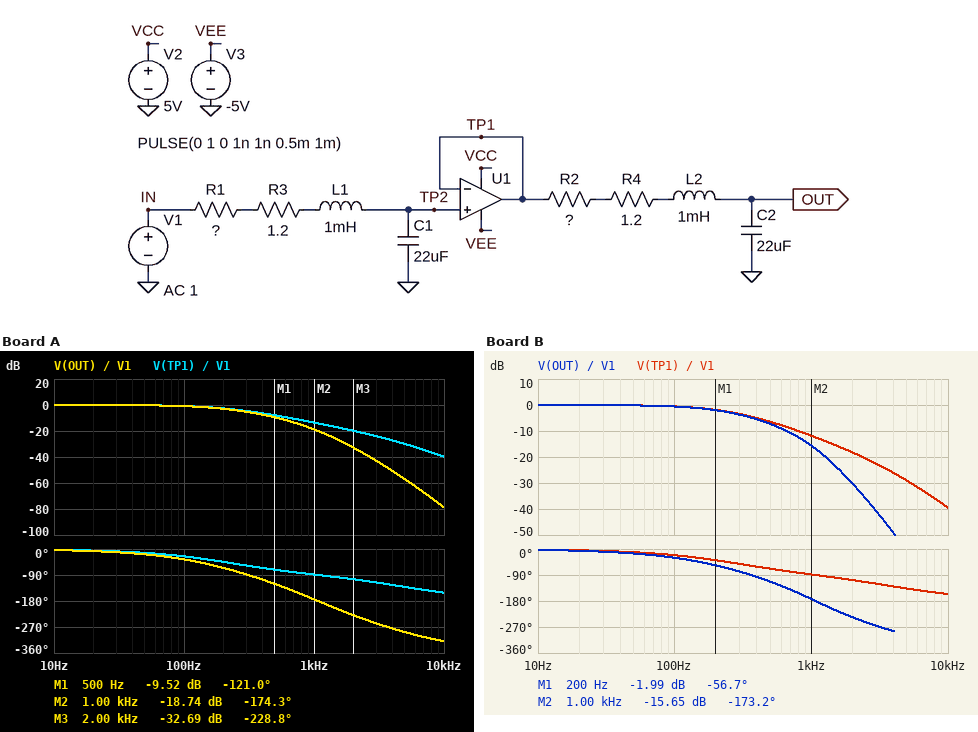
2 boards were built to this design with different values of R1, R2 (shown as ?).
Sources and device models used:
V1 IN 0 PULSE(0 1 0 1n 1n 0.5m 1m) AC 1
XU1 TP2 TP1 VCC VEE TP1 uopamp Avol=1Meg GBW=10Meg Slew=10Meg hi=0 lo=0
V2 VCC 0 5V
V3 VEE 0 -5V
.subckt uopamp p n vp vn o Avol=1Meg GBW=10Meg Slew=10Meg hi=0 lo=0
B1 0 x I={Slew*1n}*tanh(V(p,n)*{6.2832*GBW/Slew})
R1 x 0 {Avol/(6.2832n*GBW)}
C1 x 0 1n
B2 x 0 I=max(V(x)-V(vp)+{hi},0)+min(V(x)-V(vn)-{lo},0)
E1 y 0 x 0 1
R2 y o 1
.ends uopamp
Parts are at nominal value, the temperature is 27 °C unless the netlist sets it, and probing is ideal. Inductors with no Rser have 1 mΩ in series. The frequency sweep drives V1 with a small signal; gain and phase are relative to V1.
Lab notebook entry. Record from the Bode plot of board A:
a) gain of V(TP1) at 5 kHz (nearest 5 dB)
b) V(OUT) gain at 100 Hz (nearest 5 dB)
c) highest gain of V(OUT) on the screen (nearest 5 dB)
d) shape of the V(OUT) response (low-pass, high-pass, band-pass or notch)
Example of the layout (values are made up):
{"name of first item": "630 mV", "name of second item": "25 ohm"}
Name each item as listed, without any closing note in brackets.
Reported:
{"gain of V(TP1) at 5 kHz": "-30 dB", "V(OUT) gain at 100 Hz": "0 dB", "highest gain of V(OUT) on the screen": "0 dB", "shape of the V(OUT) response": "low-pass"}
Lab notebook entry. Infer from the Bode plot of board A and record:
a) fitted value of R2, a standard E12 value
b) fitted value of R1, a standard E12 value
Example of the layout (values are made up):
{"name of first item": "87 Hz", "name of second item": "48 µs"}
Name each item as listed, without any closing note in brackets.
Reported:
{"fitted value of R2, a standard E12 value": "12 Ω", "fitted value of R1, a standard E12 value": "33 Ω"}
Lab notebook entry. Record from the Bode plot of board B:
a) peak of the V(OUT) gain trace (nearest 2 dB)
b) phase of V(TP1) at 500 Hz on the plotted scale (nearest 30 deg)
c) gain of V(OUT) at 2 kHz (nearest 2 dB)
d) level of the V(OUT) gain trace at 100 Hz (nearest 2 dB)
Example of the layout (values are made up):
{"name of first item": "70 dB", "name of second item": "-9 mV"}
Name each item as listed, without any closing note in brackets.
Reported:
{"peak of the V(OUT) gain trace": "0 dB", "phase of V(TP1) at 500 Hz on the plotted scale": "-60 deg", "gain of V(OUT) at 2 kHz": "-30 dB", "level of the V(OUT) gain trace at 100 Hz": "0 dB"}
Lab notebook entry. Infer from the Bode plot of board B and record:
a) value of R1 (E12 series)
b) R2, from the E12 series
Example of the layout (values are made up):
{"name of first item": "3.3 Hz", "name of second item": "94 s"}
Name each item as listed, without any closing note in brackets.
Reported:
{"value of R1": "27 Ω", "R2, from the E12 series": "10 Ω"}
